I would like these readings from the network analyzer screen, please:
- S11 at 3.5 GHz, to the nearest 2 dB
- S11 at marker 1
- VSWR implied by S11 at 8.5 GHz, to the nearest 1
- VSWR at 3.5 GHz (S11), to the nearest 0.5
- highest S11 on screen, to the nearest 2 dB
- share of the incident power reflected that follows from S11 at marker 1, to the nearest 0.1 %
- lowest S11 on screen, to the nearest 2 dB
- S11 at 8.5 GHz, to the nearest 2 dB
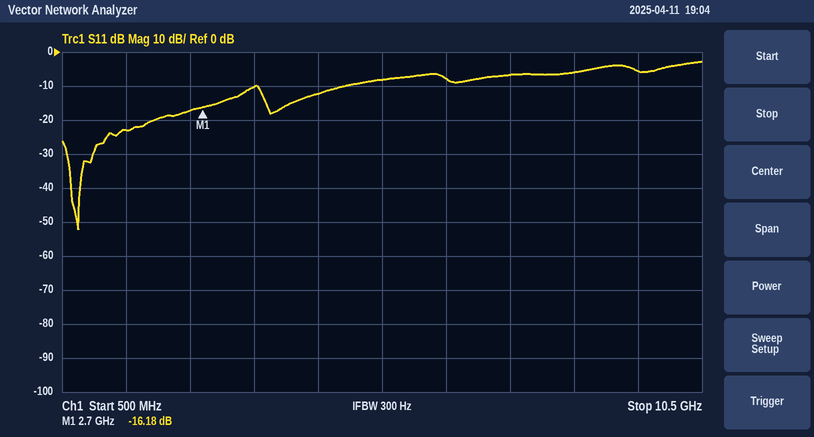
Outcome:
-10 dB
-16.18 dB
3
2.0
-2 dB
2.4 %
-52 dB
-6 dB
